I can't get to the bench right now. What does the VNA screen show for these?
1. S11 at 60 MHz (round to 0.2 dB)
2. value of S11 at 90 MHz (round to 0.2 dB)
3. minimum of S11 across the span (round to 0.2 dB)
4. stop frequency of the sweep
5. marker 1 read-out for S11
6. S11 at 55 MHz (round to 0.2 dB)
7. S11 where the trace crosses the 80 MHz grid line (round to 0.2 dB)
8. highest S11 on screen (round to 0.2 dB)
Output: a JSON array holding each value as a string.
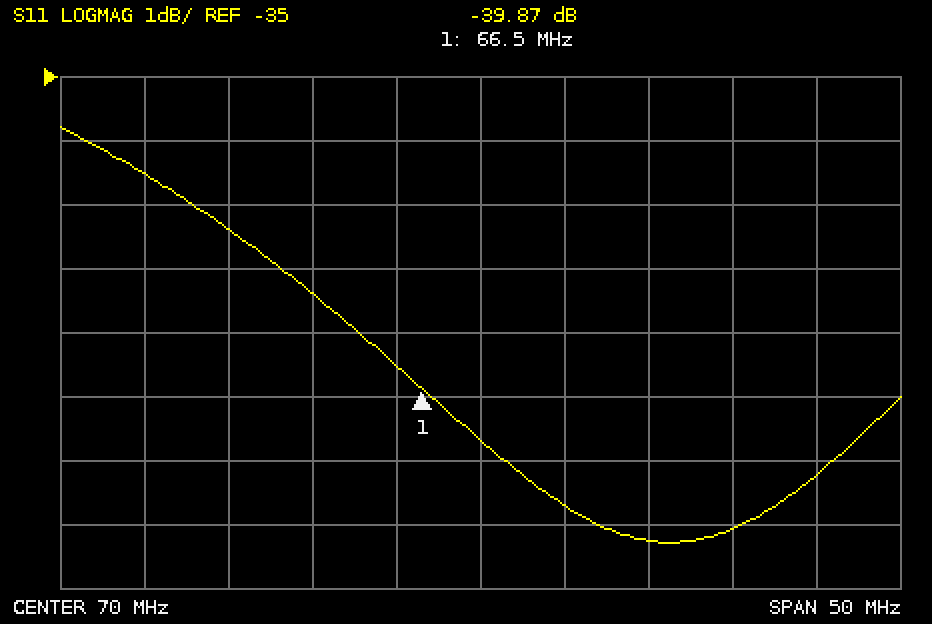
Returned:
["-38.4 dB", "-41.2 dB", "-42.2 dB", "95 MHz", "-39.87 dB", "-37.4 dB", "-42.2 dB", "-35.8 dB"]
